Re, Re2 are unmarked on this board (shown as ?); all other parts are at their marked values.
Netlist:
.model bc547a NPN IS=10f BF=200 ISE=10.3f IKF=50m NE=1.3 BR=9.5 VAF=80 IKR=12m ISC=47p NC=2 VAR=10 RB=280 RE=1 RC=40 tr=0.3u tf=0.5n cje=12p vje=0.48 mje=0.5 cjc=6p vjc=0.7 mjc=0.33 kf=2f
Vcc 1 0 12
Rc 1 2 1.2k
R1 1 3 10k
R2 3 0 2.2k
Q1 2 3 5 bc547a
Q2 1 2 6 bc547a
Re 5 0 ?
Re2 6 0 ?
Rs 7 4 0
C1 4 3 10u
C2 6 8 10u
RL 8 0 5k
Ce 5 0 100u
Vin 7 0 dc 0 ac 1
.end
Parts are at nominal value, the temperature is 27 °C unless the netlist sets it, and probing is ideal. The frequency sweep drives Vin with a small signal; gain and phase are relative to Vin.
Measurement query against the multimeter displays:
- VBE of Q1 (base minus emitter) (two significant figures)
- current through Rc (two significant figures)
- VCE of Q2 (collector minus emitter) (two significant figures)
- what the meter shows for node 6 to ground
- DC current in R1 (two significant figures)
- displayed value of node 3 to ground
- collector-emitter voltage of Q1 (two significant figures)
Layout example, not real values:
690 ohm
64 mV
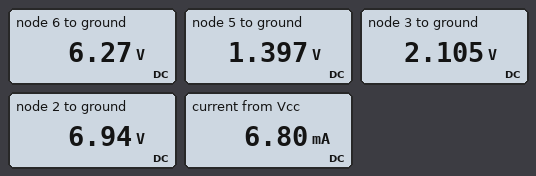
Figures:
710 mV
4.2 mA
5.7 V
6.27 V
990 µA
2.105 V
5.5 V
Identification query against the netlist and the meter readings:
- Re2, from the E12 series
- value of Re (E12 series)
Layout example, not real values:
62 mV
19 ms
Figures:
3.9 kΩ
330 Ω
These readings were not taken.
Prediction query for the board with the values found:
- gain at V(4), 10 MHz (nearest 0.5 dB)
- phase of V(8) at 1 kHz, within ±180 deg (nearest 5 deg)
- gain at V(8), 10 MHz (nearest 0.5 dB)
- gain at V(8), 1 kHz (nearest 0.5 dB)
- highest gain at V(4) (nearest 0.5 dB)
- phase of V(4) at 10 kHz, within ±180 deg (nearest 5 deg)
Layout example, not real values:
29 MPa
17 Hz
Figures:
0 dB
-170 deg
23.0 dB
41.0 dB
0 dB
0 deg
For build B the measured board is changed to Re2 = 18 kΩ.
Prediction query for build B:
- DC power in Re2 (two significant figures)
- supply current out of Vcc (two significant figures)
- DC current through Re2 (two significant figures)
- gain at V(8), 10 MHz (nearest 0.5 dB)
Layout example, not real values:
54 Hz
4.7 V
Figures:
2.2 mW
5.5 mA
350 µA
22.5 dB
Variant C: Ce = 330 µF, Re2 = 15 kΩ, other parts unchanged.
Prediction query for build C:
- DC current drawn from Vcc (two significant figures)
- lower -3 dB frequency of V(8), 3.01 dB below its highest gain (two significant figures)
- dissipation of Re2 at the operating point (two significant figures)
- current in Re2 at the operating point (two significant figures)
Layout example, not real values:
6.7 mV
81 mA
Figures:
5.6 mA
63 Hz
2.7 mW
420 µA
